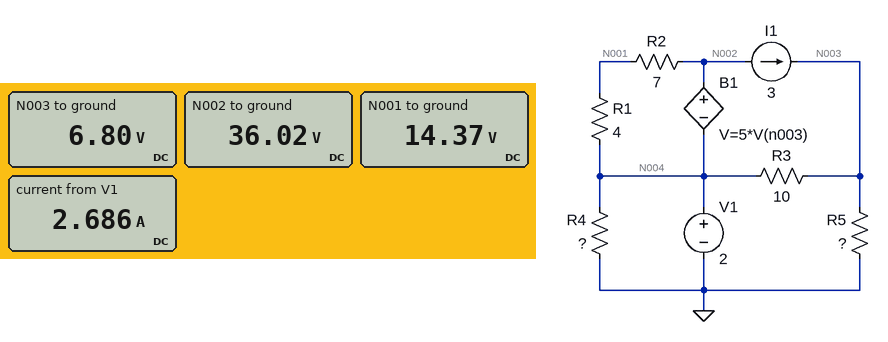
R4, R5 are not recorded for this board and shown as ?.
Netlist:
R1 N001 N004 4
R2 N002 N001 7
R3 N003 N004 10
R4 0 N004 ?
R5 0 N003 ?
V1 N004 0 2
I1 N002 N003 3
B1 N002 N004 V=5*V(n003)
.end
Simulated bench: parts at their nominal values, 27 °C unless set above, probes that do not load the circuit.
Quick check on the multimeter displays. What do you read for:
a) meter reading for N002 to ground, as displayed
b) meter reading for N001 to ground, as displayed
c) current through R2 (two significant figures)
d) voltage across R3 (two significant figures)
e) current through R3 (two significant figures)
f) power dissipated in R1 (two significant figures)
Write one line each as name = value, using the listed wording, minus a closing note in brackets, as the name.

meter reading for N002 to ground, as displayed = 36.02 V
meter reading for N001 to ground, as displayed = 14.37 V
current through R2 = 3.1 A
voltage across R3 = 4.8 V
current through R3 = 480 mA
power dissipated in R1 = 38 W
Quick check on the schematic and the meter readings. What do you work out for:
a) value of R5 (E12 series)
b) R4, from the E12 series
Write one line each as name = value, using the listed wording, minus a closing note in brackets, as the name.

value of R5 = 2.7 Ω
R4, from the E12 series = 12 Ω
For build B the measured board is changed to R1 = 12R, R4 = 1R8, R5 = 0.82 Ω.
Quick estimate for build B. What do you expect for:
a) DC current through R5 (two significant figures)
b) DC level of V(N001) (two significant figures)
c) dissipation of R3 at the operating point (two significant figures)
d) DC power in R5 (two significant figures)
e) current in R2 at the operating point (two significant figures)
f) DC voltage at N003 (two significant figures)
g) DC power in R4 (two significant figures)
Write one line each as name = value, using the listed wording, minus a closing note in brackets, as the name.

DC current through R5 = 3.0 A
DC level of V(N001) = 9.7 V
dissipation of R3 at the operating point = 18 mW
DC power in R5 = 7.2 W
current in R2 at the operating point = 640 mA
DC voltage at N003 = 2.4 V
DC power in R4 = 2.2 W
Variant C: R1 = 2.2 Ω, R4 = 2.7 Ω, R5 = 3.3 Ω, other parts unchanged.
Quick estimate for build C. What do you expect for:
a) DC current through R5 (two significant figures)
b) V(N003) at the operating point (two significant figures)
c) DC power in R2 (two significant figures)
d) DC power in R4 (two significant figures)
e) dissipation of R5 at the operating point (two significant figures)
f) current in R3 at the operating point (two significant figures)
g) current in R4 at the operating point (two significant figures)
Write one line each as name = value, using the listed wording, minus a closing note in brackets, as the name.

DC current through R5 = 2.4 A
V(N003) at the operating point = 7.9 V
DC power in R2 = 130 W
DC power in R4 = 1.5 W
dissipation of R5 at the operating point = 19 W
current in R3 at the operating point = 590 mA
current in R4 at the operating point = 740 mA
